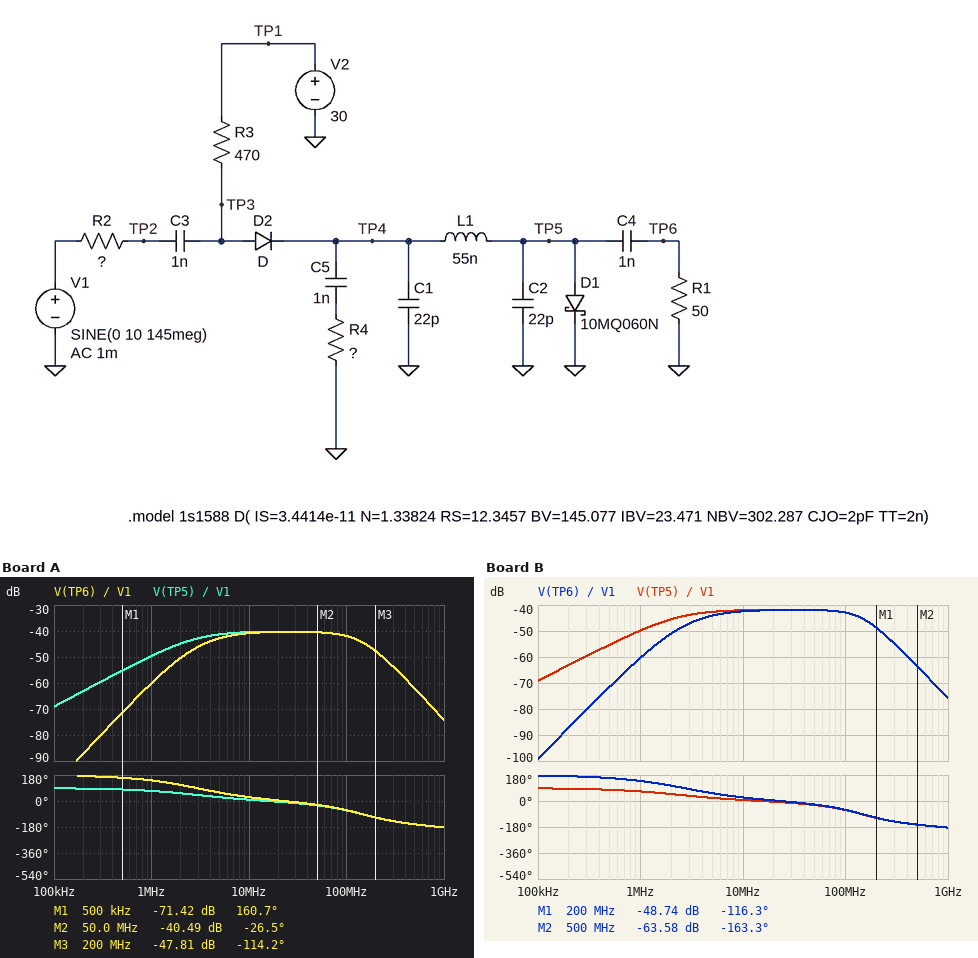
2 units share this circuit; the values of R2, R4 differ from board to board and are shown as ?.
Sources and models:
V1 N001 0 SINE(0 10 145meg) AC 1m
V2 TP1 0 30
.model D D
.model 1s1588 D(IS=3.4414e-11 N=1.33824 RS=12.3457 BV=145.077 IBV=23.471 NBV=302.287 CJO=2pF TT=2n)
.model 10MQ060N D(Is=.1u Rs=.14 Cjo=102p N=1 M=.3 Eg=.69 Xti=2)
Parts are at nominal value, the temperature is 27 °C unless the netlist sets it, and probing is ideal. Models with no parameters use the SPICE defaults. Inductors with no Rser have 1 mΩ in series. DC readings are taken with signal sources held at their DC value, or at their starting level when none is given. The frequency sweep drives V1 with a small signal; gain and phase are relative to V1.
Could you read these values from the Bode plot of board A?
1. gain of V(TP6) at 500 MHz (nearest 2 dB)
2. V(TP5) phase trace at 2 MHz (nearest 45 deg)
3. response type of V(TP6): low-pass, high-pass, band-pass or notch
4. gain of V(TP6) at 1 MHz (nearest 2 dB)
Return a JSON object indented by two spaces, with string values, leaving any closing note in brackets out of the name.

{
  "gain of V(TP6) at 500 MHz": "-62 dB",
  "V(TP5) phase trace at 2 MHz": "45 deg",
  "response type of V(TP6): low-pass, high-pass, band-pass or notch": "band-pass",
  "gain of V(TP6) at 1 MHz": "-60 dB"
}
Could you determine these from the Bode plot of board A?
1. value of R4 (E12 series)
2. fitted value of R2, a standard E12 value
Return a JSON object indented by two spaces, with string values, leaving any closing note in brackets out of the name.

{
  "value of R4": "82 Ω",
  "fitted value of R2, a standard E12 value": "56 Ω"
}
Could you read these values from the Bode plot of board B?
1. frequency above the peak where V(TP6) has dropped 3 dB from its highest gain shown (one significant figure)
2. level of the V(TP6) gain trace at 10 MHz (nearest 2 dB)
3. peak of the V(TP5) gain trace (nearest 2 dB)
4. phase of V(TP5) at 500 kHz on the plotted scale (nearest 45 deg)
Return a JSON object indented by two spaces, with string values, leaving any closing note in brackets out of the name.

{
  "frequency above the peak where V(TP6) has dropped 3 dB from its highest gain shown": "100 MHz",
  "level of the V(TP6) gain trace at 10 MHz": "-42 dB",
  "peak of the V(TP5) gain trace": "-42 dB",
  "phase of V(TP5) at 500 kHz on the plotted scale": "90 deg"
}
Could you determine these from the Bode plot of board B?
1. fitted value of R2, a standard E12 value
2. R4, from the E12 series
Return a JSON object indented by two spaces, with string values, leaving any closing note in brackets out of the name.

{
  "fitted value of R2, a standard E12 value": "68 Ω",
  "R4, from the E12 series": "82 Ω"
}
